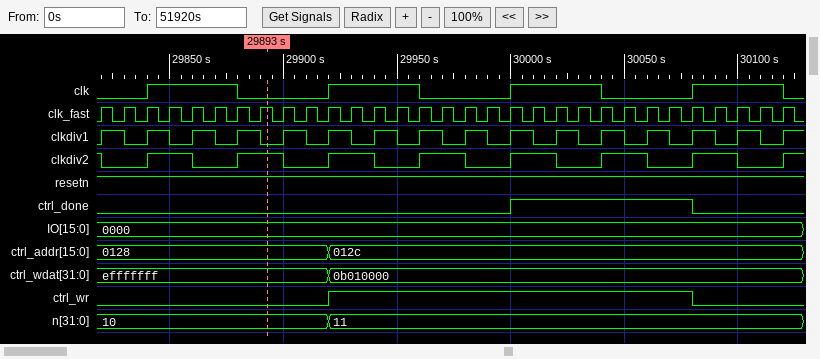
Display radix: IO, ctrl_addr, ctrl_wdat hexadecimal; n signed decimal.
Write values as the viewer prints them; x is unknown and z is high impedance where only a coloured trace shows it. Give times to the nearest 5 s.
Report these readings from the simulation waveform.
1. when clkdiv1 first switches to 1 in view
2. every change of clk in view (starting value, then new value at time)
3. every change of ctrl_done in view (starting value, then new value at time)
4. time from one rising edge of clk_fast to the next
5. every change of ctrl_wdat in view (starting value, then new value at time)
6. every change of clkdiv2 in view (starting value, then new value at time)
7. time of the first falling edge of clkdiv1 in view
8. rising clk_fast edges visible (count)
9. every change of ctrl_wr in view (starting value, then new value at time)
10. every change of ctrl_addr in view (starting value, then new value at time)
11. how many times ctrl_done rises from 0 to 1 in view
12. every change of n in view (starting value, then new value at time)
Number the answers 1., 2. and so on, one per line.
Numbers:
1. 29820 s
2. 0, 1 at 29840 s, 0 at 29880 s, 1 at 29920 s, 0 at 29960 s, 1 at 30000 s, 0 at 30040 s, 1 at 30080 s, 0 at 30120 s
3. 0, 1 at 30000 s, 0 at 30080 s
4. 10 s
5. efffffff, 0b010000 at 29920 s
6. 1, 0 at 29820 s, 1 at 29840 s, 0 at 29860 s, 1 at 29880 s, 0 at 29900 s, 1 at 29920 s, 0 at 29940 s, 1 at 29960 s, 0 at 29980 s, 1 at 30000 s, 0 at 30020 s, 1 at 30040 s, 0 at 30060 s, 1 at 30080 s, 0 at 30100 s, 1 at 30120 s
7. 29830 s
8. 31
9. 0, 1 at 29920 s, 0 at 30080 s
10. 0128, 012c at 29920 s
11. 1
12. 10, 11 at 29920 s
